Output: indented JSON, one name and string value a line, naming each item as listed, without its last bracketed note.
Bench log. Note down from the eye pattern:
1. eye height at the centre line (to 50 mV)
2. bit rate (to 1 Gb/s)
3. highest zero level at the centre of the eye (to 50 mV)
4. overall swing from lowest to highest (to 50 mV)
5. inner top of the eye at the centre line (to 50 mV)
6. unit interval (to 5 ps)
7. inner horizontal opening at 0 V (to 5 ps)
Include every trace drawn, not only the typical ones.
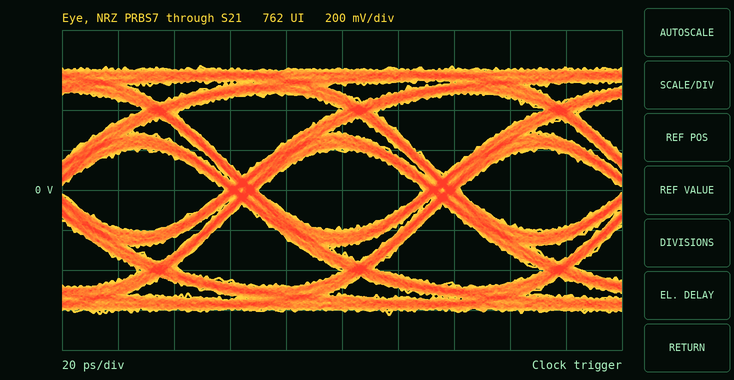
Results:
{
  "eye height at the centre line": "400 mV",
  "bit rate": "14 Gb/s",
  "highest zero level at the centre of the eye": "-200 mV",
  "overall swing from lowest to highest": "1.25 V",
  "inner top of the eye at the centre line": "200 mV",
  "unit interval": "70 ps",
  "inner horizontal opening at 0 V": "60 ps"
}
